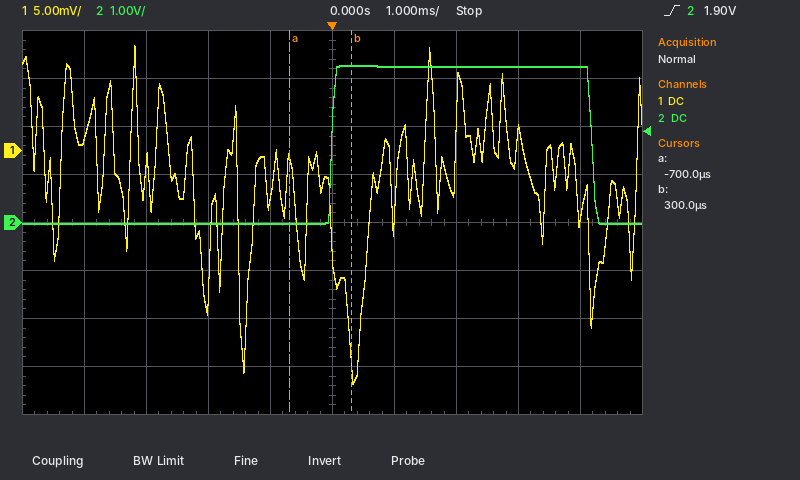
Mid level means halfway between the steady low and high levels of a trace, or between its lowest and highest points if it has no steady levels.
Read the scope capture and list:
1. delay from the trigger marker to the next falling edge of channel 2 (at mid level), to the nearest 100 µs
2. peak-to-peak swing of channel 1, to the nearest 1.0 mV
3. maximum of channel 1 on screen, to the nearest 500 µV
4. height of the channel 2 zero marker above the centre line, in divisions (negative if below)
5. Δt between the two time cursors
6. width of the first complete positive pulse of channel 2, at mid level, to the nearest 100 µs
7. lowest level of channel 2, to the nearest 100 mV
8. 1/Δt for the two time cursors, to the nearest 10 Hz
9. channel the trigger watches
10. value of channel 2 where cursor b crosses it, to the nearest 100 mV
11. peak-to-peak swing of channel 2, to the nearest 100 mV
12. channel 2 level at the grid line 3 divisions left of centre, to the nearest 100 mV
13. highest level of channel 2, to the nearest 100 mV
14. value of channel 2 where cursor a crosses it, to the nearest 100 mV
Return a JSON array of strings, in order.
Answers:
["4.2 ms", "35.0 mV", "11.0 mV", "0.0 div", "1.0 ms", "4.2 ms", "0.0 V", "1.00 kHz", "channel 2", "3.3 V", "3.3 V", "0.0 V", "3.3 V", "0.0 V"]
